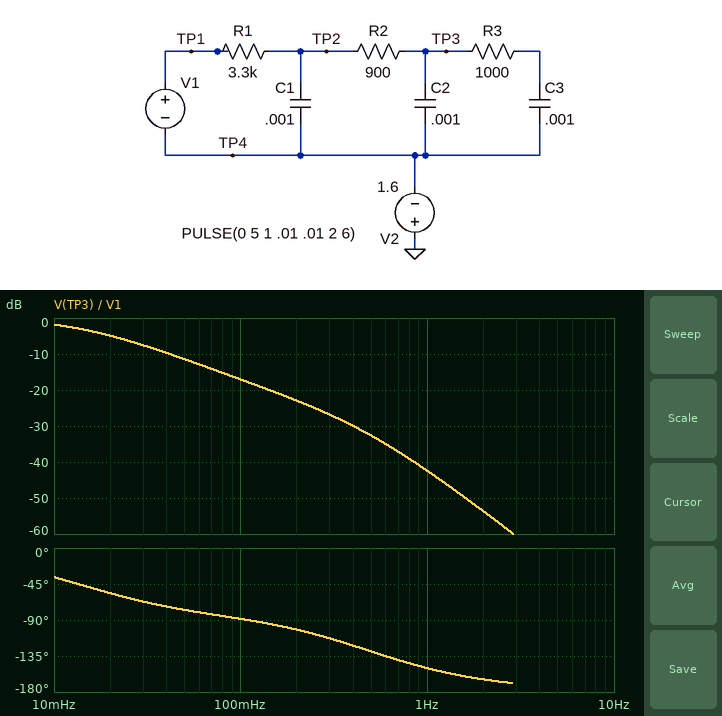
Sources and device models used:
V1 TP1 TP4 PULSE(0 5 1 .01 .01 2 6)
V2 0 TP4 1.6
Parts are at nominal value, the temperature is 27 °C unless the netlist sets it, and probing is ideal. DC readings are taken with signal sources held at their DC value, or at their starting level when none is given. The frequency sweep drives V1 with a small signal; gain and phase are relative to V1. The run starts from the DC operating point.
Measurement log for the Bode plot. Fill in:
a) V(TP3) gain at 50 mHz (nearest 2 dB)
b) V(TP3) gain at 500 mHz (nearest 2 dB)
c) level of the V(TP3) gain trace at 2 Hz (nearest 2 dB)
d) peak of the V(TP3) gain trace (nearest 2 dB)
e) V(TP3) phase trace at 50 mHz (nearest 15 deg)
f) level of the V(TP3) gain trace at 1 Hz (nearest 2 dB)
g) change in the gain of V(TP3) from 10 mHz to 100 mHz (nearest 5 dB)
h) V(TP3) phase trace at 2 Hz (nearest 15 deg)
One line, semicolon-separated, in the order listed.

-12 dB; -32 dB; -54 dB; -2 dB; -75 deg; -42 dB; -15 dB; -165 deg
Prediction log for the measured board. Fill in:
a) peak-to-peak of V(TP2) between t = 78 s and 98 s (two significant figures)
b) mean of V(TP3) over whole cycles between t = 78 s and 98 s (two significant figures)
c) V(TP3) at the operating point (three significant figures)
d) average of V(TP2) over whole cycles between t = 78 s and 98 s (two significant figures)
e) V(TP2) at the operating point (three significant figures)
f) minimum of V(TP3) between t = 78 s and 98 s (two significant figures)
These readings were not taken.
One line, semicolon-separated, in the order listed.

1.2 V; 74 mV; -1.60 V; 74 mV; -1.60 V; -190 mV
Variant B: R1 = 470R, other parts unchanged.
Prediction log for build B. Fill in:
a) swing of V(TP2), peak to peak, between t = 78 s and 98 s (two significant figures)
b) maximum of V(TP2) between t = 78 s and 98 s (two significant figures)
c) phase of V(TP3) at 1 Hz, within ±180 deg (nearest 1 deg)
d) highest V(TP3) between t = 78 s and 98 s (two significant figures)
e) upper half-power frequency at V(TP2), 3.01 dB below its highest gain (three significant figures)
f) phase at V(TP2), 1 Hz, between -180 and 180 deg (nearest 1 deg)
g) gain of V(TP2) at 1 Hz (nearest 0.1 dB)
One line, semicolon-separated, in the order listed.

3.9 V; 2.6 V; -136 deg; 1.3 V; 126 mHz; -64 deg; -10.6 dB
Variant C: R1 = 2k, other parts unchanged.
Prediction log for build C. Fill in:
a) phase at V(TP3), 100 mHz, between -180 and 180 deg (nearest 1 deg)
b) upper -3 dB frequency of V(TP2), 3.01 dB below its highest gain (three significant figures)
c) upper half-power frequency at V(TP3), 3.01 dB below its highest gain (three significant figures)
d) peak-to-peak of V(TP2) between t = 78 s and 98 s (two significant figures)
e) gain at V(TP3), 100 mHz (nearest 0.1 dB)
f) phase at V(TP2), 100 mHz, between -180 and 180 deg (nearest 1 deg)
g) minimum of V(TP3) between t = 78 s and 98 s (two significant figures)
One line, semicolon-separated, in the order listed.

-83 deg; 22.7 mHz; 20.7 mHz; 1.8 V; -13.5 dB; -45 deg; -330 mV
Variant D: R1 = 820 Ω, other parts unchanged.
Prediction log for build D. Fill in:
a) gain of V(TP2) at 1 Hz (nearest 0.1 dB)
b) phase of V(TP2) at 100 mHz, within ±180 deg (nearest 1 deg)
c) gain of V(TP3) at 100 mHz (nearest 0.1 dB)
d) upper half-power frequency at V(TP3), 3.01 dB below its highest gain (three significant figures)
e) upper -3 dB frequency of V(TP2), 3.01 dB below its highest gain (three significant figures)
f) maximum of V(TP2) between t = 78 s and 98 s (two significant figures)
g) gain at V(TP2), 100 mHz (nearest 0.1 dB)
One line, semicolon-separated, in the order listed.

-15.0 dB; -31 deg; -8.6 dB; 37.4 mHz; 55.0 mHz; 2.1 V; -4.6 dB
